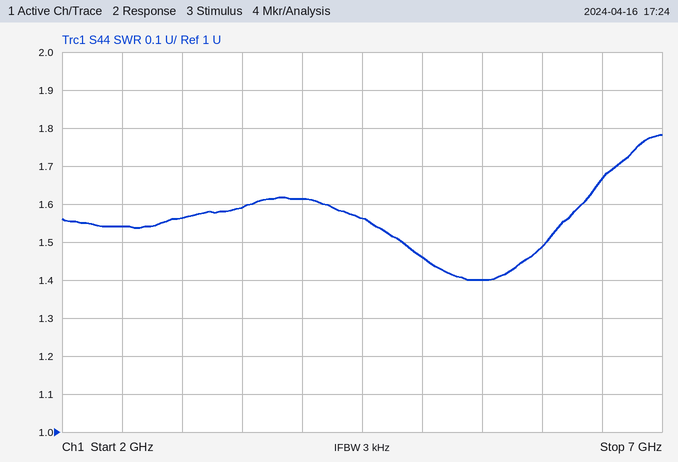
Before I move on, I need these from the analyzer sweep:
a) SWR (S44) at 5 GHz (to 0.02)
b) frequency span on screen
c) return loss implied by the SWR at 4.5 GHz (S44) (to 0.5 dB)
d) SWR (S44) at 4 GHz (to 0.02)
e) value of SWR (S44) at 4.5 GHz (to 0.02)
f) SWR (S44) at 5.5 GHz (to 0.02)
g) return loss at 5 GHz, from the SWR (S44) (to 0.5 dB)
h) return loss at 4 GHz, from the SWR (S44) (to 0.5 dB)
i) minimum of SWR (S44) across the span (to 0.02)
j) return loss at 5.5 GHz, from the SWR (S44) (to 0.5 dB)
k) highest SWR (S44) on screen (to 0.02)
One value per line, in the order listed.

1.46
5 GHz
13.0 dB
1.62
1.56
1.40
14.5 dB
12.5 dB
1.40
15.5 dB
1.78
